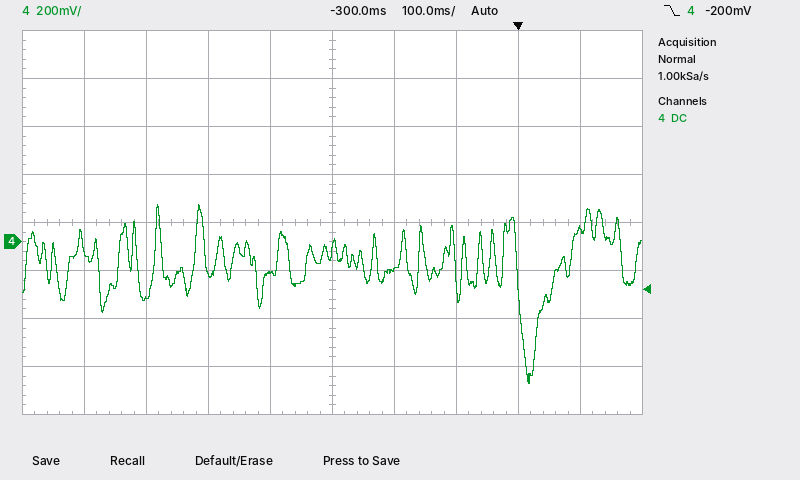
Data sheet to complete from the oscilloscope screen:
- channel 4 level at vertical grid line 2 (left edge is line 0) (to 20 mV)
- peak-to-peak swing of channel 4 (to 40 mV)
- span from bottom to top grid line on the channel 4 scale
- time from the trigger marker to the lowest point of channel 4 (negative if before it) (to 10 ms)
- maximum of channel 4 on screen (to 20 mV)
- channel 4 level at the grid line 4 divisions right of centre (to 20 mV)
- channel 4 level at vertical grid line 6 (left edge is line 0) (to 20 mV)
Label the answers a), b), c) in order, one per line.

a) -240 mV
b) 760 mV
c) 1.6 V
d) +20 ms
e) 160 mV
f) 60 mV
g) -120 mV
